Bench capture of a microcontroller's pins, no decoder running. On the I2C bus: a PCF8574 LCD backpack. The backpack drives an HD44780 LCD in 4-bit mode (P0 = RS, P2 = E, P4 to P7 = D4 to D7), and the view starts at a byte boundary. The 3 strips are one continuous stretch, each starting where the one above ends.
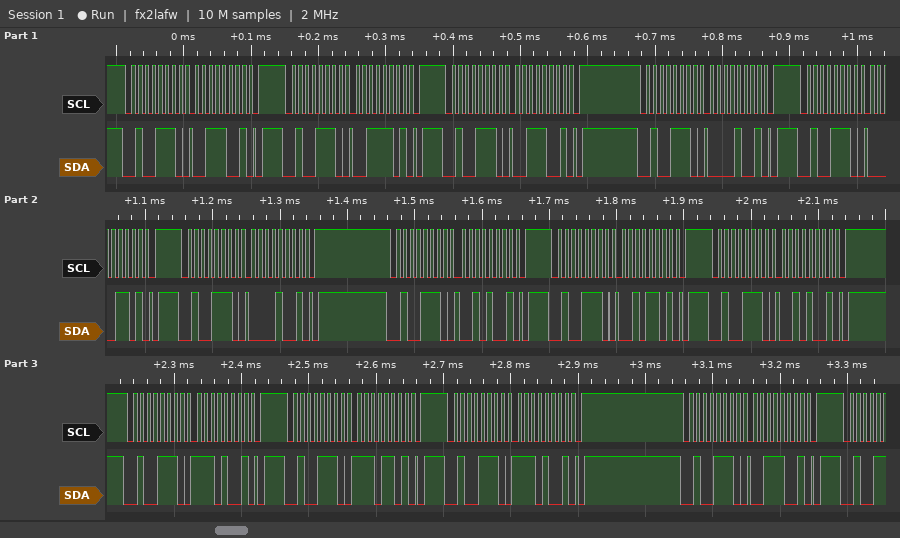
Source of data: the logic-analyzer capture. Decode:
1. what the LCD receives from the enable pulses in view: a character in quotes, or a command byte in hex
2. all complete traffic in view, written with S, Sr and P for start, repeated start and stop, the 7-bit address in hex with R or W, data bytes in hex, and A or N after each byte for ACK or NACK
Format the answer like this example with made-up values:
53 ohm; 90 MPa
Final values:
'0' '.'; S 27W A 39 A P S 27W A 3D A P S 27W A 39 A P S 27W A 09 A P S 27W A 0D A P S 27W A 09 A P S 27W A 29 A P S 27W A 2D A P S 27W A 29 A P S 27W A E9 A P S 27W A ED A P S 27W A E9 A P S 27W A 39 A P
